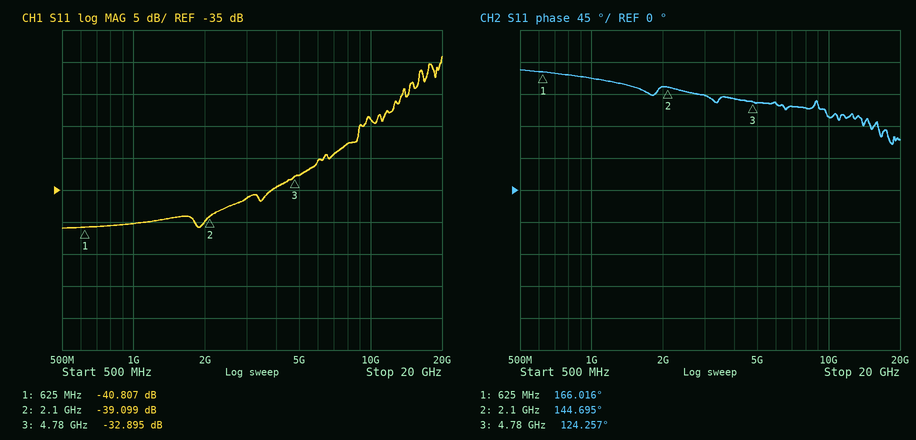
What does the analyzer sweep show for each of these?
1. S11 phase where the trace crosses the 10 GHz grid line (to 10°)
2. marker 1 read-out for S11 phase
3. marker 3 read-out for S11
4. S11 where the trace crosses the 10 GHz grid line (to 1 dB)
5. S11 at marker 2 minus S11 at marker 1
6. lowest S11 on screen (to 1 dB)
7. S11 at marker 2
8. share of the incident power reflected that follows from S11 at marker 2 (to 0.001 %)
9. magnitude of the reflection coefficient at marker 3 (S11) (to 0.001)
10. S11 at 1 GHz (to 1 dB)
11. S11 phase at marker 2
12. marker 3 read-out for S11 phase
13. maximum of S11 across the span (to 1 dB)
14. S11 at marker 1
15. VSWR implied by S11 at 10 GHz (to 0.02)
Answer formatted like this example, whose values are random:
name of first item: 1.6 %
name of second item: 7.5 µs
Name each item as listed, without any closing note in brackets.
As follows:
S11 phase where the trace crosses the 10 GHz grid line: 100°
marker 1 read-out for S11 phase: 166.016°
marker 3 read-out for S11: -32.895 dB
S11 where the trace crosses the 10 GHz grid line: -24 dB
S11 at marker 2 minus S11 at marker 1: 1.708 dB
lowest S11 on screen: -41 dB
S11 at marker 2: -39.099 dB
share of the incident power reflected that follows from S11 at marker 2: 0.012 %
magnitude of the reflection coefficient at marker 3 (S11): 0.023
S11 at 1 GHz: -40 dB
S11 phase at marker 2: 144.695°
marker 3 read-out for S11 phase: 124.257°
maximum of S11 across the span: -14 dB
S11 at marker 1: -40.807 dB
VSWR implied by S11 at 10 GHz: 1.14
